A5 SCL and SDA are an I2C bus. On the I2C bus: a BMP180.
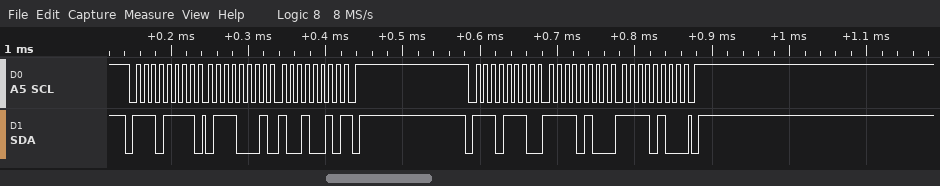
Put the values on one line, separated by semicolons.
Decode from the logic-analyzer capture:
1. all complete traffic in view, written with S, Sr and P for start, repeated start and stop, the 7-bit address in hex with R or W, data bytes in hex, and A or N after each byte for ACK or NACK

S 77R A 71 A 92 N P S 77W A F4 A F4 A P
